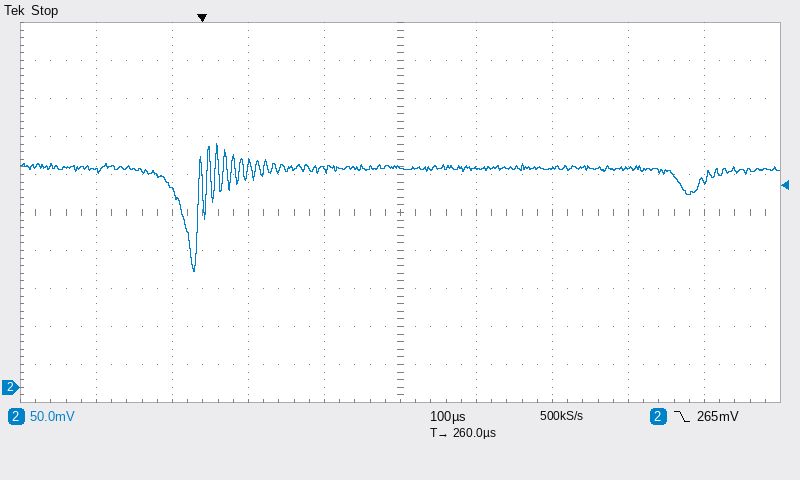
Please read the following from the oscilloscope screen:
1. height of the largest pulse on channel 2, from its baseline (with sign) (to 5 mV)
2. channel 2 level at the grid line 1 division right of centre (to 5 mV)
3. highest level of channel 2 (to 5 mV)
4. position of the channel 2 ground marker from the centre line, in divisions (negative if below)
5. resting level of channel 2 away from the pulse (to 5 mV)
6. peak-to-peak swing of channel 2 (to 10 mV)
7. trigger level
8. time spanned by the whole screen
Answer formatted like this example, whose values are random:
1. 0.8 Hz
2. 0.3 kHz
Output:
1. -135 mV
2. 290 mV
3. 320 mV
4. -4.6 div
5. 290 mV
6. 170 mV
7. 265 mV
8. 1 ms
